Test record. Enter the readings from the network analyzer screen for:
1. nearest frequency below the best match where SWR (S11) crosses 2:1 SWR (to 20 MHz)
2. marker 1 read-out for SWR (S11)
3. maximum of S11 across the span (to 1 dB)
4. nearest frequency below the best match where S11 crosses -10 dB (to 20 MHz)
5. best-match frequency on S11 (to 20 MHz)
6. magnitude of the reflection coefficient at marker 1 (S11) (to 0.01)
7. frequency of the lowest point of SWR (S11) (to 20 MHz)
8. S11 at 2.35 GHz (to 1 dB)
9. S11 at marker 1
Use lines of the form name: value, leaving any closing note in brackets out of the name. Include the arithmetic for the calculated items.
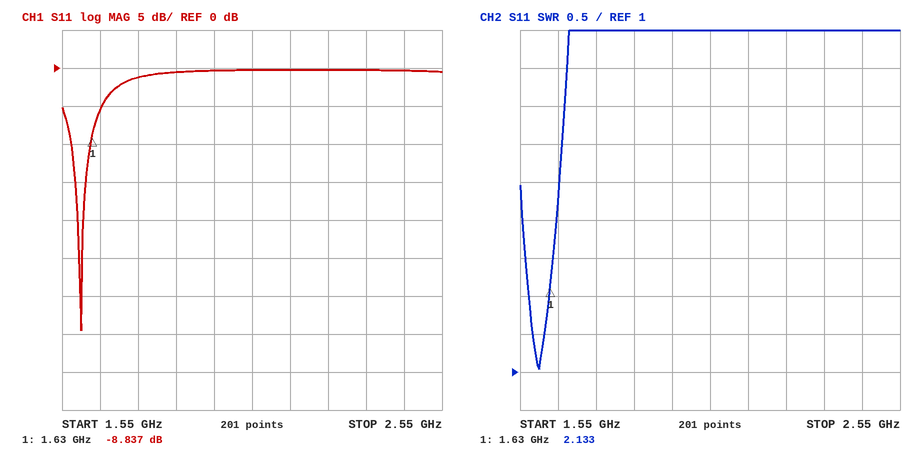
nearest frequency below the best match where SWR (S11) crosses 2:1 SWR: 1.58 GHz
marker 1 read-out for SWR: 2.133
maximum of S11 across the span: 0 dB
nearest frequency below the best match where S11 crosses -10 dB: 1.58 GHz
best-match frequency on S11: 1.60 GHz
magnitude of the reflection coefficient at marker 1 (S11): 10^(-8.837/20) ≈ 0.36
frequency of the lowest point of SWR (S11): 1.60 GHz
S11 at 2.35 GHz: 0 dB
S11 at marker 1: -8.837 dB
